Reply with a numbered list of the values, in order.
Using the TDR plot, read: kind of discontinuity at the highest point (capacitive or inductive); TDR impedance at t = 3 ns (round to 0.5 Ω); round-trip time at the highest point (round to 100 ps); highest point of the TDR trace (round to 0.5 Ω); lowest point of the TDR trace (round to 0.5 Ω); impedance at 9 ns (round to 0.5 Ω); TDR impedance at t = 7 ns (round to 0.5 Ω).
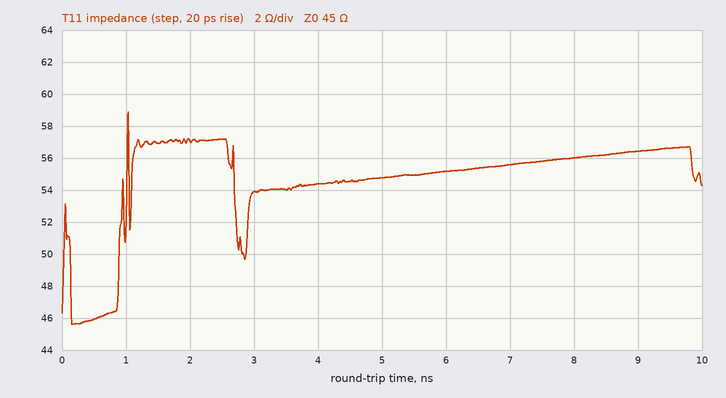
1. inductive
2. 54.0 Ω
3. 1.0 ns
4. 59.0 Ω
5. 45.5 Ω
6. 56.5 Ω
7. 55.5 Ω
